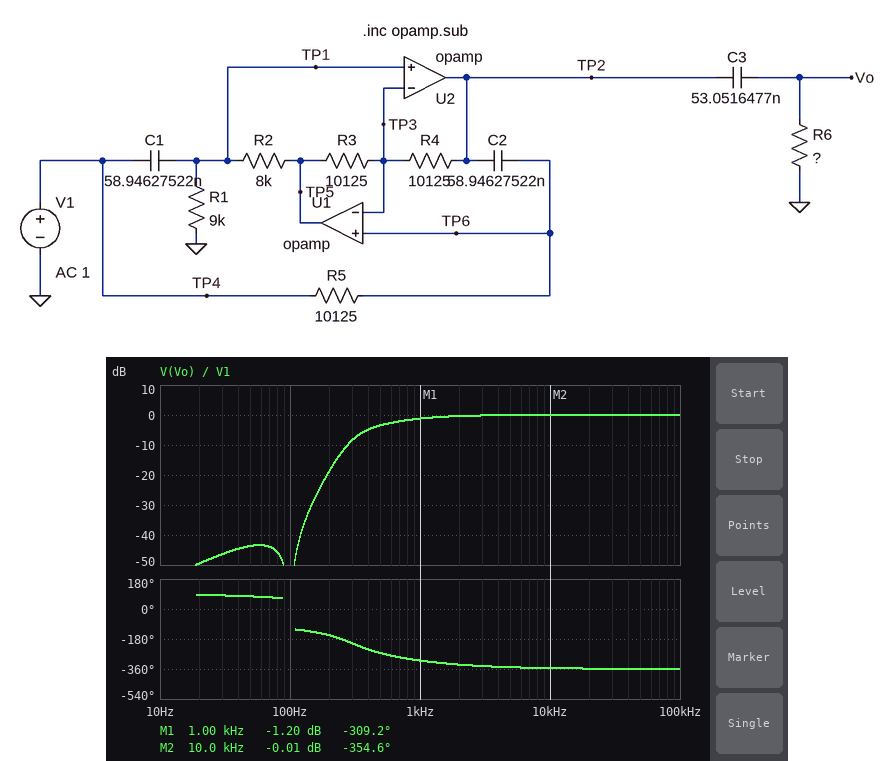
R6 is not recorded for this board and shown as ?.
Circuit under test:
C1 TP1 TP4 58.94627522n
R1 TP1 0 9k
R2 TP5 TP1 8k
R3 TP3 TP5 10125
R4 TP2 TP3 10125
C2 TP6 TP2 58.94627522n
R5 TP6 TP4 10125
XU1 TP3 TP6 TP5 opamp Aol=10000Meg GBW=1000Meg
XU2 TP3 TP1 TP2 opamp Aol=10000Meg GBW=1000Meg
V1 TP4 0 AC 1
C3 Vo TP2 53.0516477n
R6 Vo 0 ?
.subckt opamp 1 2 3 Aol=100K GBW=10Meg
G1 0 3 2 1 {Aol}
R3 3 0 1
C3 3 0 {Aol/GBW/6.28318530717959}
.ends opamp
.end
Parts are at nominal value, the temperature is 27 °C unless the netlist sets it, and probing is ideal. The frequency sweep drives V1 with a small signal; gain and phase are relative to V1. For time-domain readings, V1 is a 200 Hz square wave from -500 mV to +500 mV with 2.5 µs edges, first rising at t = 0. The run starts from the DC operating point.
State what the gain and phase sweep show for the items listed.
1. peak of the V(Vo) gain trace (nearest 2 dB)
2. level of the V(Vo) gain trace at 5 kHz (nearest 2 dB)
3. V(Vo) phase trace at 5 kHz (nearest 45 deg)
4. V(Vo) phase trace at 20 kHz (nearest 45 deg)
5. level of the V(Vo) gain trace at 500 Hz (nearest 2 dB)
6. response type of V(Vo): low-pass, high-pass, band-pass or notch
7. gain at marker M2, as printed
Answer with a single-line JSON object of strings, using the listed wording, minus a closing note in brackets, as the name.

{"peak of the V(Vo) gain trace": "0 dB", "level of the V(Vo) gain trace at 5 kHz": "0 dB", "V(Vo) phase trace at 5 kHz": "-360 deg", "V(Vo) phase trace at 20 kHz": "-360 deg", "level of the V(Vo) gain trace at 500 Hz": "-4 dB", "response type of V(Vo): low-pass, high-pass, band-pass or notch": "high-pass", "gain at marker M2, as printed": "-0.01 dB"}
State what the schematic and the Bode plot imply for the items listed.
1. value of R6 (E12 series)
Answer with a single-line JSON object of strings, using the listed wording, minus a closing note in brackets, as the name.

{"value of R6": "4.7 kΩ"}
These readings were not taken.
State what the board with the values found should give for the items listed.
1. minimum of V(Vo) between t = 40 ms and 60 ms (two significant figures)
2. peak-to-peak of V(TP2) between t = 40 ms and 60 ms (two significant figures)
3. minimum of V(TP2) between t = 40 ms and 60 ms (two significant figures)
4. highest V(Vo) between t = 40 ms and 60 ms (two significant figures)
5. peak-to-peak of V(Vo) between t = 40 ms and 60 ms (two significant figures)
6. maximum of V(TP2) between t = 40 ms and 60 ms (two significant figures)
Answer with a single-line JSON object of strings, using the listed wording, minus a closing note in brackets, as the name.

{"minimum of V(Vo) between t = 40 ms and 60 ms": "-930 mV", "peak-to-peak of V(TP2) between t = 40 ms and 60 ms": "1.9 V", "minimum of V(TP2) between t = 40 ms and 60 ms": "-930 mV", "highest V(Vo) between t = 40 ms and 60 ms": "930 mV", "peak-to-peak of V(Vo) between t = 40 ms and 60 ms": "1.9 V", "maximum of V(TP2) between t = 40 ms and 60 ms": "930 mV"}
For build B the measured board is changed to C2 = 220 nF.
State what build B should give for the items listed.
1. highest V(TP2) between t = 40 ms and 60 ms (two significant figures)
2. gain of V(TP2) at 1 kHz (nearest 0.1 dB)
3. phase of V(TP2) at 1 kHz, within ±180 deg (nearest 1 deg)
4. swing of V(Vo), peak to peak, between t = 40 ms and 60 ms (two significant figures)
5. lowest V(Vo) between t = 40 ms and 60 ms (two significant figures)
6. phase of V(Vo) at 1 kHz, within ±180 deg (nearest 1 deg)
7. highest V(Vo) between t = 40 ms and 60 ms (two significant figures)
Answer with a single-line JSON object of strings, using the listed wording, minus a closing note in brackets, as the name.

{"highest V(TP2) between t = 40 ms and 60 ms": "1.1 V", "gain of V(TP2) at 1 kHz": "-0.2 dB", "phase of V(TP2) at 1 kHz, within ±180 deg": "17 deg", "swing of V(Vo), peak to peak, between t = 40 ms and 60 ms": "2.0 V", "lowest V(Vo) between t = 40 ms and 60 ms": "-990 mV", "phase of V(Vo) at 1 kHz, within ±180 deg": "50 deg", "highest V(Vo) between t = 40 ms and 60 ms": "990 mV"}
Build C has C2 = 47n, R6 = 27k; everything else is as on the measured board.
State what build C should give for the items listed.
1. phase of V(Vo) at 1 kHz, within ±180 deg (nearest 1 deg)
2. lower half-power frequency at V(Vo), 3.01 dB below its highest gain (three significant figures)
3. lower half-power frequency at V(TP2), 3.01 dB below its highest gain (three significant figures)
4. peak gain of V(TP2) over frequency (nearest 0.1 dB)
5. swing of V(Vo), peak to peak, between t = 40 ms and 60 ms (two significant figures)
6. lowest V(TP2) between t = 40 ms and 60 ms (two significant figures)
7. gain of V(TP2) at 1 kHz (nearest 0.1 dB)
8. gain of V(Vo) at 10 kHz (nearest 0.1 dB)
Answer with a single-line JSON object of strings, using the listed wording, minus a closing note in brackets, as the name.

{"phase of V(Vo) at 1 kHz, within ±180 deg": "25 deg", "lower half-power frequency at V(Vo), 3.01 dB below its highest gain": "305 Hz", "lower half-power frequency at V(TP2), 3.01 dB below its highest gain": "299 Hz", "peak gain of V(TP2) over frequency": "1.4 dB", "swing of V(Vo), peak to peak, between t = 40 ms and 60 ms": "1.7 V", "lowest V(TP2) between t = 40 ms and 60 ms": "-880 mV", "gain of V(TP2) at 1 kHz": "0.5 dB", "gain of V(Vo) at 10 kHz": "0 dB"}
